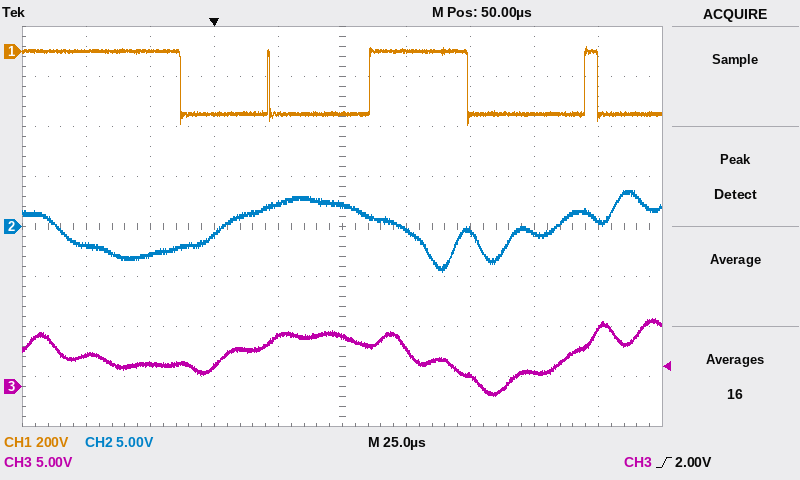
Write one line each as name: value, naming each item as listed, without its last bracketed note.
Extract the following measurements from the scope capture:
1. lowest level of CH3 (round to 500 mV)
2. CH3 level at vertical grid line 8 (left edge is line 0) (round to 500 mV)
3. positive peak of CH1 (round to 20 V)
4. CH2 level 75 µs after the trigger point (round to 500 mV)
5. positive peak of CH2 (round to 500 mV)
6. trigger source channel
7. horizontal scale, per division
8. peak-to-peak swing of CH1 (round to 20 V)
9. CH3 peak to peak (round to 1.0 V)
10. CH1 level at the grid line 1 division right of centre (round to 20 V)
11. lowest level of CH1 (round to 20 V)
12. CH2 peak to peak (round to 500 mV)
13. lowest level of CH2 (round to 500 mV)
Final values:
lowest level of CH3: -1.0 V
CH3 level at vertical grid line 8 (left edge is line 0): 1.5 V
positive peak of CH1: 20 V
CH2 level 75 µs after the trigger point: -500 mV
positive peak of CH2: 3.5 V
trigger source channel: CH3
horizontal scale, per division: 25 µs
peak-to-peak swing of CH1: 320 V
CH3 peak to peak: 8.0 V
CH1 level at the grid line 1 division right of centre: 0 V
lowest level of CH1: -300 V
CH2 peak to peak: 8.0 V
lowest level of CH2: -4.5 V
